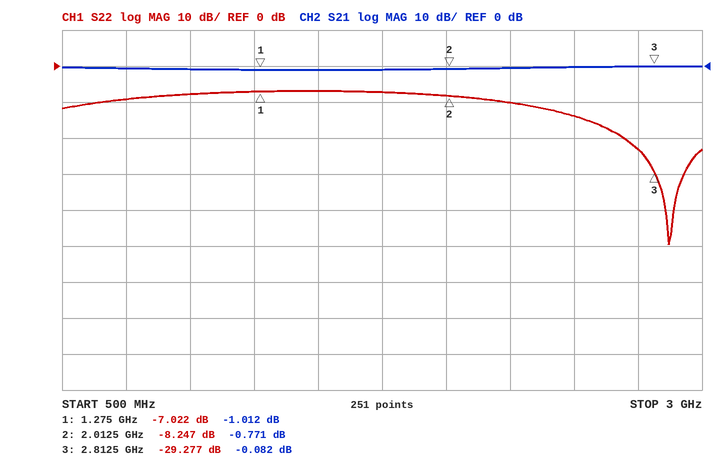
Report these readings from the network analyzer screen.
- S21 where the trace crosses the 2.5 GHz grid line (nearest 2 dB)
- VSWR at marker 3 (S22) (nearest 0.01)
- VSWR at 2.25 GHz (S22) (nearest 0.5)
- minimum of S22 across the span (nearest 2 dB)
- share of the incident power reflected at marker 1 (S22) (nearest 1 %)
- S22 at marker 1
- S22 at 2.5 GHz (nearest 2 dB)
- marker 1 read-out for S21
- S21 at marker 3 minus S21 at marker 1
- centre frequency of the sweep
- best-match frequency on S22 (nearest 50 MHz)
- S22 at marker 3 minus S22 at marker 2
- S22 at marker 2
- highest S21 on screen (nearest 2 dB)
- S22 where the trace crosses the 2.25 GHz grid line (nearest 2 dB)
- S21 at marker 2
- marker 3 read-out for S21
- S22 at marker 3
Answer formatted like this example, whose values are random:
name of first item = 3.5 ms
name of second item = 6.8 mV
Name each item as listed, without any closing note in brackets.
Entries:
S21 where the trace crosses the 2.5 GHz grid line = 0 dB
VSWR at marker 3 (S22) = 1.07
VSWR at 2.25 GHz (S22) = 2.0
minimum of S22 across the span = -50 dB
share of the incident power reflected at marker 1 (S22) = 20 %
S22 at marker 1 = -7.022 dB
S22 at 2.5 GHz = -14 dB
marker 1 read-out for S21 = -1.012 dB
S21 at marker 3 minus S21 at marker 1 = 0.930 dB
centre frequency of the sweep = 1.75 GHz
best-match frequency on S22 = 2.85 GHz
S22 at marker 3 minus S22 at marker 2 = -21.030 dB
S22 at marker 2 = -8.247 dB
highest S21 on screen = 0 dB
S22 where the trace crosses the 2.25 GHz grid line = -10 dB
S21 at marker 2 = -0.771 dB
marker 3 read-out for S21 = -0.082 dB
S22 at marker 3 = -29.277 dB
